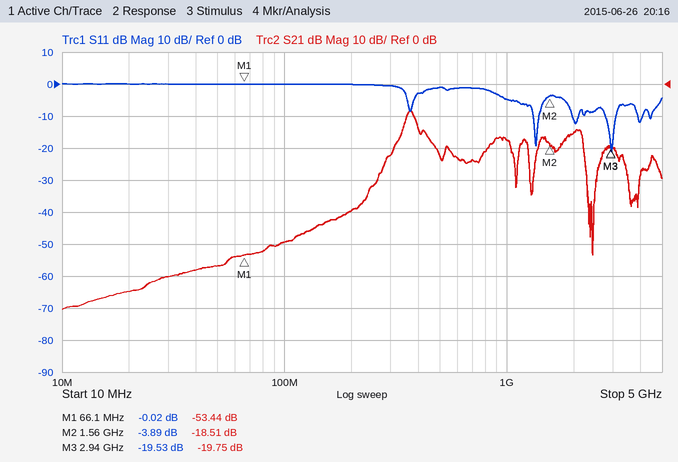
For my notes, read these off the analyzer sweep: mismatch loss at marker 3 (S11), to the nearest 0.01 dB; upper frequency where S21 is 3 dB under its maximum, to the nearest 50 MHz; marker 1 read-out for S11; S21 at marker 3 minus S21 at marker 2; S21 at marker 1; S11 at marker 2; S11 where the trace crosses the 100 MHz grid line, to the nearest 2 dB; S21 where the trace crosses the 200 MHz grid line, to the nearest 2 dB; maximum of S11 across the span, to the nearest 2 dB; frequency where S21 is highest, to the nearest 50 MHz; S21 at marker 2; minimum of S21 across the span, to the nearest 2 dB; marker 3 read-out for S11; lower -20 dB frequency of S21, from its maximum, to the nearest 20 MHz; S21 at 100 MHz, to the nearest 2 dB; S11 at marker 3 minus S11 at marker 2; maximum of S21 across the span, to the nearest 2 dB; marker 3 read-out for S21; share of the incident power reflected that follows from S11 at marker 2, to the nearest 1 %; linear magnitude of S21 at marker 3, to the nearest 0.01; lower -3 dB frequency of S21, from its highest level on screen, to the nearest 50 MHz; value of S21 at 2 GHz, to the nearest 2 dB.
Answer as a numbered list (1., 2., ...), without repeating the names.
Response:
1. 0.05 dB
2. 400 MHz
3. -0.02 dB
4. -1.24 dB
5. -53.44 dB
6. -3.89 dB
7. 0 dB
8. -40 dB
9. 0 dB
10. 350 MHz
11. -18.51 dB
12. -70 dB
13. -19.53 dB
14. 260 MHz
15. -50 dB
16. -15.64 dB
17. -8 dB
18. -19.75 dB
19. 41 %
20. 0.10
21. 350 MHz
22. -16 dB
